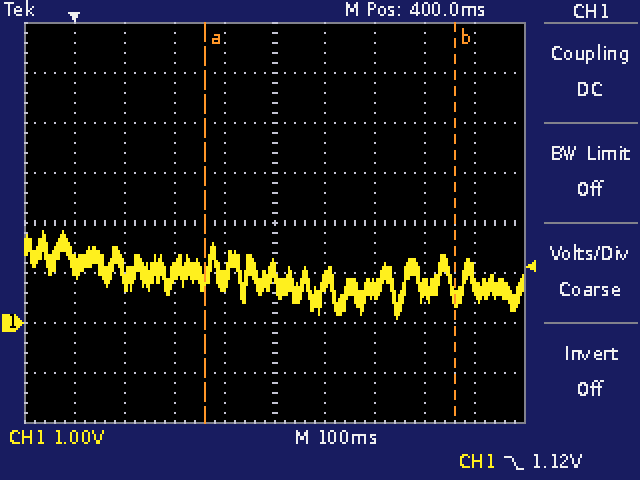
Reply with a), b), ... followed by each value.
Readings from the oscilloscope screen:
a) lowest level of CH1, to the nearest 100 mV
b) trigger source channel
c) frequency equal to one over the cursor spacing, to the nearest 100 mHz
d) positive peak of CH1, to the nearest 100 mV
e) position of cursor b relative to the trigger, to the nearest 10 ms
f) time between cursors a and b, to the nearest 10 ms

a) 100 mV
b) CH1
c) 2.0 Hz
d) 1.8 V
e) +760 ms
f) 500 ms
